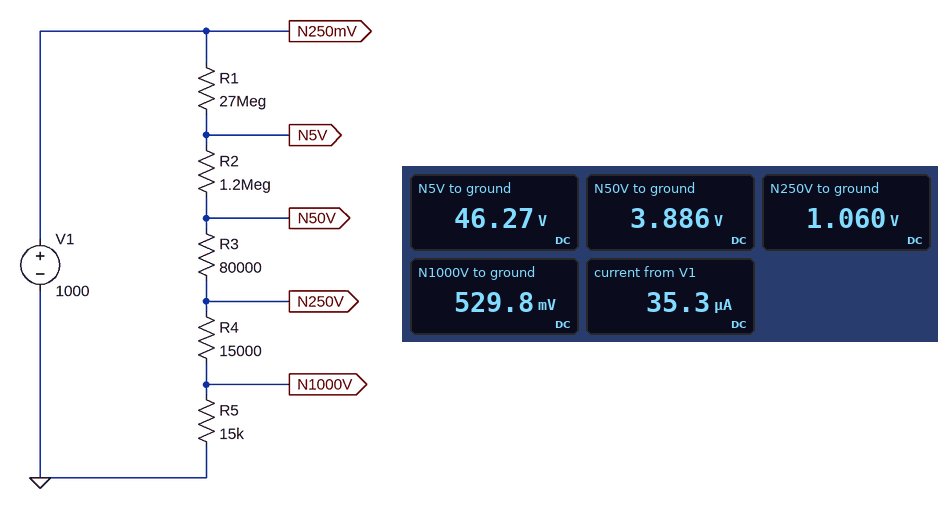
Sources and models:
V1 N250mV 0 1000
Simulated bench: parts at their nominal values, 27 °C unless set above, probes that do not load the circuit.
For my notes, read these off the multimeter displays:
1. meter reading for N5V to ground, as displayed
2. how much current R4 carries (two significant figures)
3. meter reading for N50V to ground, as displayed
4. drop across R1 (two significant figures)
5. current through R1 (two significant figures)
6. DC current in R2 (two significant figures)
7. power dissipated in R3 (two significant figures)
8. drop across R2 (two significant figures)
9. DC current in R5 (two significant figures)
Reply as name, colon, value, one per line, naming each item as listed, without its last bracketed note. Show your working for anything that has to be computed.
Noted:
meter reading for N5V to ground, as displayed: 46.27 V
how much current R4 carries: (1.06 V - 529.8 mV) / 15 kΩ = 35 µA
meter reading for N50V to ground, as displayed: 3.886 V
drop across R1: 1 kV - 46.27 V = 950 V
current through R1: (1 kV - 46.27 V) / 27 MΩ = 35 µA
DC current in R2: (46.27 V - 3.886 V) / 1.2 MΩ = 35 µA
power dissipated in R3: (3.886 V - 1.06 V)^2 / 80 kΩ = 100 µW
drop across R2: 46.27 V - 3.886 V = 42 V
DC current in R5: (529.8 mV) / 15 kΩ = 35 µA
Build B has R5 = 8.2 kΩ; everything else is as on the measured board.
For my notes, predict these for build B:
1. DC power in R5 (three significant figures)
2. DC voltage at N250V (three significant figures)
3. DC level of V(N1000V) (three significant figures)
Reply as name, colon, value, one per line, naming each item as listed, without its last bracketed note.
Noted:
DC power in R5: 10.2 µW
DC voltage at N250V: 820 mV
DC level of V(N1000V): 290 mV
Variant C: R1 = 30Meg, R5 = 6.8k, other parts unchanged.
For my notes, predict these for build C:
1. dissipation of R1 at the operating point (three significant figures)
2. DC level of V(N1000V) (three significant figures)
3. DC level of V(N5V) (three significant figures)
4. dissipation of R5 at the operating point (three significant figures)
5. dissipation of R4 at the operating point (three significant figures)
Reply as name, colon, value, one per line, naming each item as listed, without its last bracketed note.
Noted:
dissipation of R1 at the operating point: 30.6 mW
DC level of V(N1000V): 217 mV
DC level of V(N5V): 41.6 V
dissipation of R5 at the operating point: 6.94 µW
dissipation of R4 at the operating point: 15.3 µW
